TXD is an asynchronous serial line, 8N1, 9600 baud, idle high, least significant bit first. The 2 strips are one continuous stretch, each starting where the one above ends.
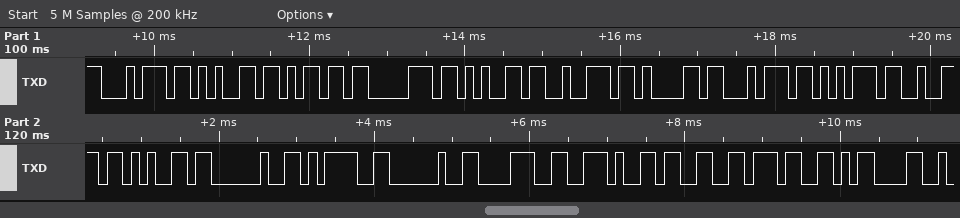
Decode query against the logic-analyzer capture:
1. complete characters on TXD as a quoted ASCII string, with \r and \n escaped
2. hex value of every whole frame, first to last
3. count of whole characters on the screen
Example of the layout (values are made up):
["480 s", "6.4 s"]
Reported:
["\"temperature = 8.37\\r\"", "74 65 6D 70 65 72 61 74 75 72 65 20 3D 20 38 2E 33 37 0D", "19"]
